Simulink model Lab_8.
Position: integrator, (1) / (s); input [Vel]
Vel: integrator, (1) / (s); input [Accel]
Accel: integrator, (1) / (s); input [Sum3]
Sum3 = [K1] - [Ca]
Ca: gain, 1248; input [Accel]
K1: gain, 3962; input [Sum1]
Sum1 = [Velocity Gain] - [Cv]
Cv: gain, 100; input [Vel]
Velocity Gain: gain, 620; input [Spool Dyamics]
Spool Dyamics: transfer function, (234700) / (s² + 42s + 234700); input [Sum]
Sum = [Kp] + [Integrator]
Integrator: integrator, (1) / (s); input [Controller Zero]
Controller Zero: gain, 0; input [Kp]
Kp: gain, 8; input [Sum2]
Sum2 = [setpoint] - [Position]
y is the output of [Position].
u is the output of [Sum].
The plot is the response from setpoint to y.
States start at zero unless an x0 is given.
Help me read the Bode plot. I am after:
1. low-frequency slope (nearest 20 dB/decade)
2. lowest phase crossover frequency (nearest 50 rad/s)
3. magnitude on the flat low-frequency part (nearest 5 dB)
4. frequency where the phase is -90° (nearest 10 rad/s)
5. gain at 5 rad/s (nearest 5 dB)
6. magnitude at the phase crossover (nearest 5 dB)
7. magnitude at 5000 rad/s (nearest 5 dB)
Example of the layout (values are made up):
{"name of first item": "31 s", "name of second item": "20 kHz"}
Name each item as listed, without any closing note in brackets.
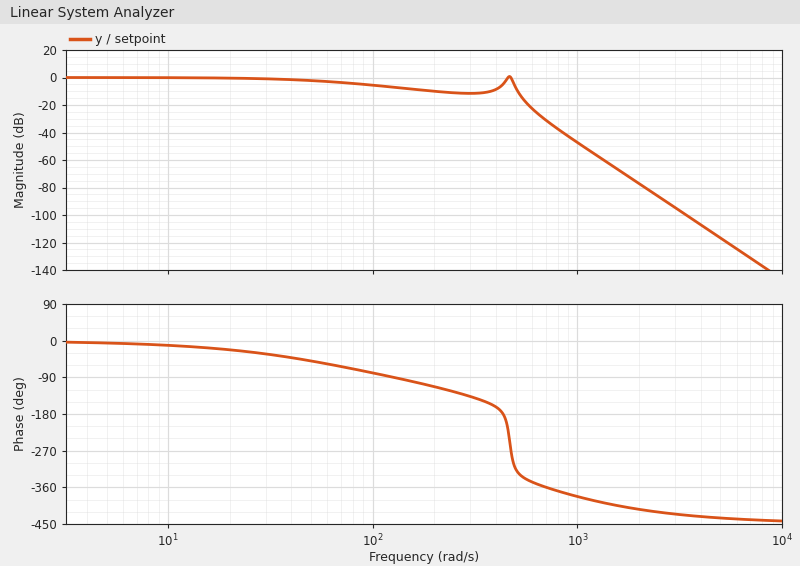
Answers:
{"low-frequency slope": "0 dB/decade", "lowest phase crossover frequency": "450 rad/s", "magnitude on the flat low-frequency part": "0 dB", "frequency where the phase is -90°": "130 rad/s", "gain at 5 rad/s": "0 dB", "magnitude at the phase crossover": "-5 dB", "magnitude at 5000 rad/s": "-115 dB"}
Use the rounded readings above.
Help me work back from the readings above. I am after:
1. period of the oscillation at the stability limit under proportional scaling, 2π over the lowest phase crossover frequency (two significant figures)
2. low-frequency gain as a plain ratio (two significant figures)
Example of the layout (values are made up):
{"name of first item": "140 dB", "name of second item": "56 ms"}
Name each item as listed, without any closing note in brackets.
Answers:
{"period of the oscillation at the stability limit under proportional scaling, 2π over the lowest phase crossover frequency": "0.014 s", "low-frequency gain as a plain ratio": "1.0"}
